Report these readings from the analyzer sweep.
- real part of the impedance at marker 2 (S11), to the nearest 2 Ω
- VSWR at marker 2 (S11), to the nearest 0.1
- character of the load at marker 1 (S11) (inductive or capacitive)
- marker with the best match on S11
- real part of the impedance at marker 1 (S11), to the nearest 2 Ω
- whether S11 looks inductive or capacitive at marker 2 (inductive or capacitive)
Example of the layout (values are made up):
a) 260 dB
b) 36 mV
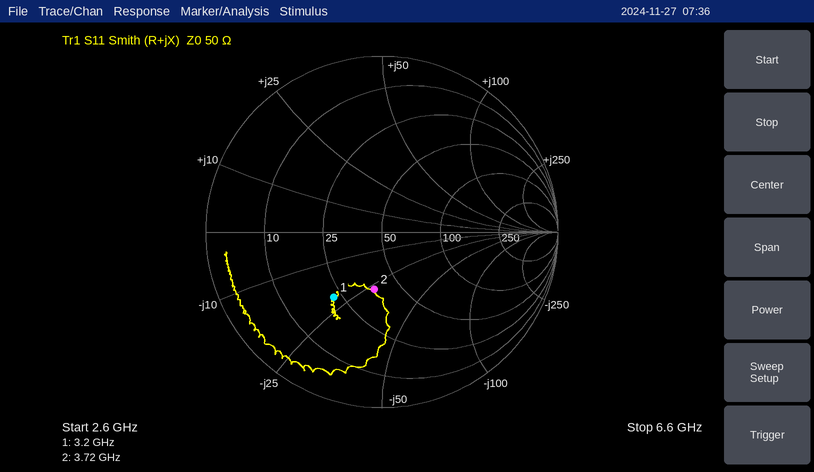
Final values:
a) 38 Ω
b) 2.0
c) capacitive
d) marker 2
e) 22 Ω
f) capacitive
